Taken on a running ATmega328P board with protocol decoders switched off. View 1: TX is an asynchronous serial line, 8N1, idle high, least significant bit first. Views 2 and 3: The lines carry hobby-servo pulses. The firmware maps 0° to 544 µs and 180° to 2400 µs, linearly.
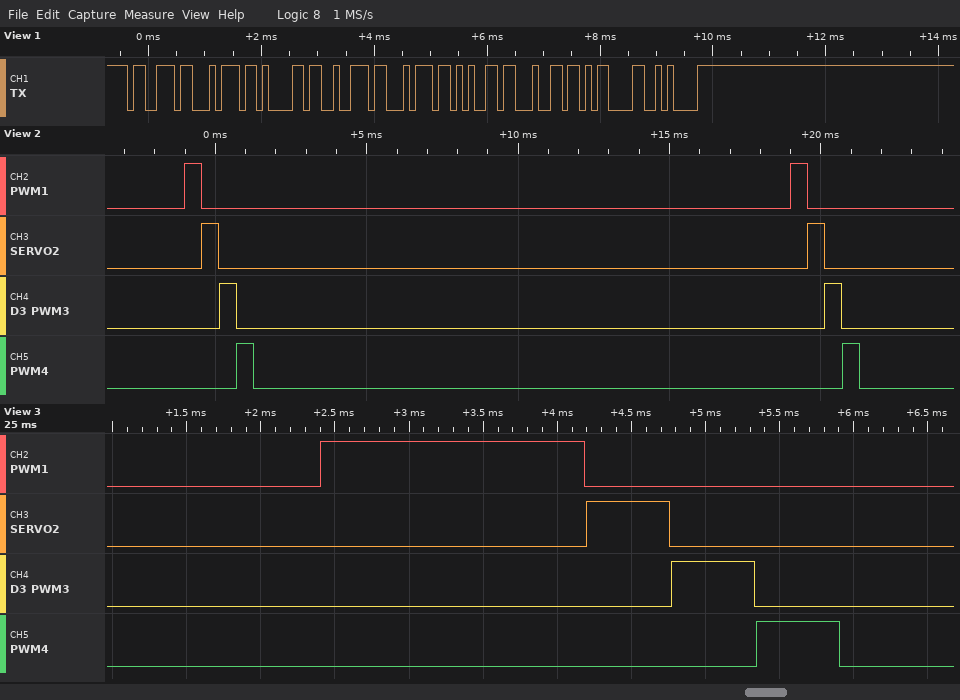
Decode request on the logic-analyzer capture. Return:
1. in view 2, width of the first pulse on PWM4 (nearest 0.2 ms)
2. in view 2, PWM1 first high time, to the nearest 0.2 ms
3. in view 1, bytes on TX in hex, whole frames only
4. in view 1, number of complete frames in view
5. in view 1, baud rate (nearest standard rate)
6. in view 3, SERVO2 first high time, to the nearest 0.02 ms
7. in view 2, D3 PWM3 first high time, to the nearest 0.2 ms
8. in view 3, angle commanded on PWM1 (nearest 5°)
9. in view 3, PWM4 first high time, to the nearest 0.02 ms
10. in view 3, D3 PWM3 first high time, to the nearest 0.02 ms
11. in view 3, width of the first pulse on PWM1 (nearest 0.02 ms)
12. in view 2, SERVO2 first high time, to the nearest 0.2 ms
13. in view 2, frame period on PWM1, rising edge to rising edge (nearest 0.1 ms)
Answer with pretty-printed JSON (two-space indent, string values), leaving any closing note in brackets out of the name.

{
  "in view 2, width of the first pulse on PWM4": "0.6 ms",
  "in view 2, PWM1 first high time, to the nearest 0.2 ms": "0.6 ms",
  "in view 1, bytes on TX in hex, whole frames only": "73 74 61 72 74 65 64 0D 0A",
  "in view 1, number of complete frames in view": "9",
  "in view 1, baud rate": "9600 baud",
  "in view 3, SERVO2 first high time, to the nearest 0.02 ms": "0.56 ms",
  "in view 2, D3 PWM3 first high time, to the nearest 0.2 ms": "0.6 ms",
  "in view 3, angle commanded on PWM1": "120°",
  "in view 3, PWM4 first high time, to the nearest 0.02 ms": "0.56 ms",
  "in view 3, D3 PWM3 first high time, to the nearest 0.02 ms": "0.56 ms",
  "in view 3, width of the first pulse on PWM1": "1.78 ms",
  "in view 2, SERVO2 first high time, to the nearest 0.2 ms": "0.6 ms",
  "in view 2, frame period on PWM1, rising edge to rising edge": "20.0 ms"
}
